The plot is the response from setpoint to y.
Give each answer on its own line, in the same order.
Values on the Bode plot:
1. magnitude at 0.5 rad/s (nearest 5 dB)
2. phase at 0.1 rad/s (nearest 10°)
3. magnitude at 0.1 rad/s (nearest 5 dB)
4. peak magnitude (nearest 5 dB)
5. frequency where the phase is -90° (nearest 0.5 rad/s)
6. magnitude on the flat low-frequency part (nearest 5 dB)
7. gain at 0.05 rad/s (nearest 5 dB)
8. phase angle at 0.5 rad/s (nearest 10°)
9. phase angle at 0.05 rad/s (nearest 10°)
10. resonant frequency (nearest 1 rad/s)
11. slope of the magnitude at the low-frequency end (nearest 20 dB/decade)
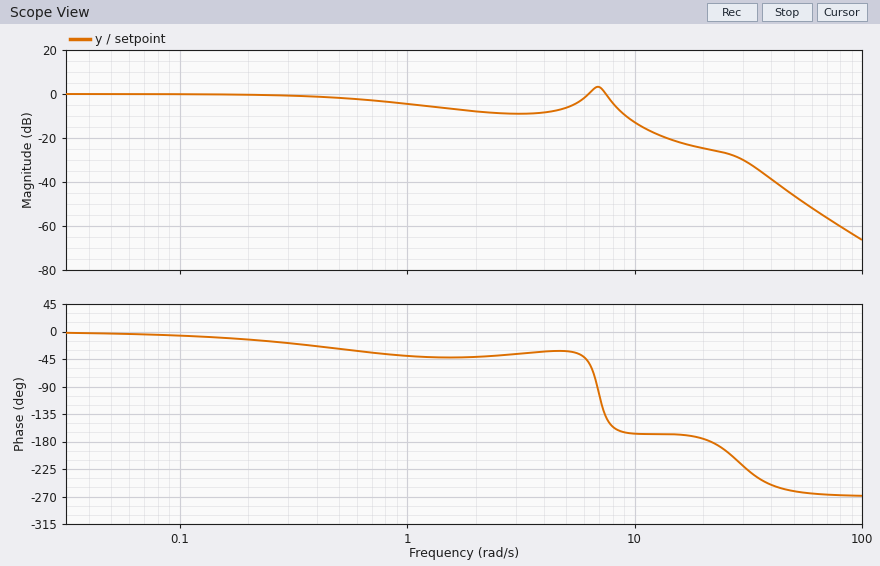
0 dB
-10°
0 dB
5 dB
7.0 rad/s
0 dB
0 dB
-30°
0°
7 rad/s
0 dB/decade
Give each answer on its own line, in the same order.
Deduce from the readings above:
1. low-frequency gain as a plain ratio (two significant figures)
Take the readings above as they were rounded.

1.0
